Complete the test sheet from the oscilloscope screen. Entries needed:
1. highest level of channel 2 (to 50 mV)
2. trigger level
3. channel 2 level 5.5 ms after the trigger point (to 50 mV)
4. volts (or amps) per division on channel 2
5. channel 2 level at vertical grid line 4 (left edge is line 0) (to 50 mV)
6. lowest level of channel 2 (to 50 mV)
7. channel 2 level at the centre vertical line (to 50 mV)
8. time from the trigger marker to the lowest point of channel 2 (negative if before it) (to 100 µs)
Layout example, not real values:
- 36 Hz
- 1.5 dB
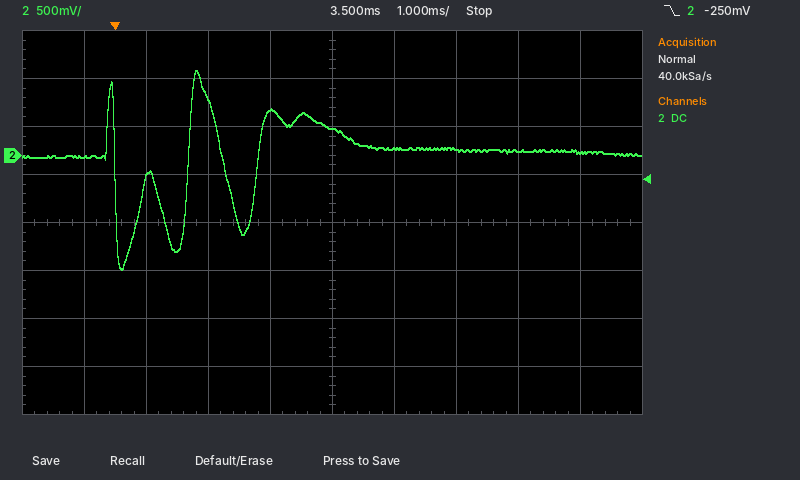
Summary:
- 900 mV
- -250 mV
- 50 mV
- 500 mV
- 450 mV
- -1.20 V
- 300 mV
- +100 µs
